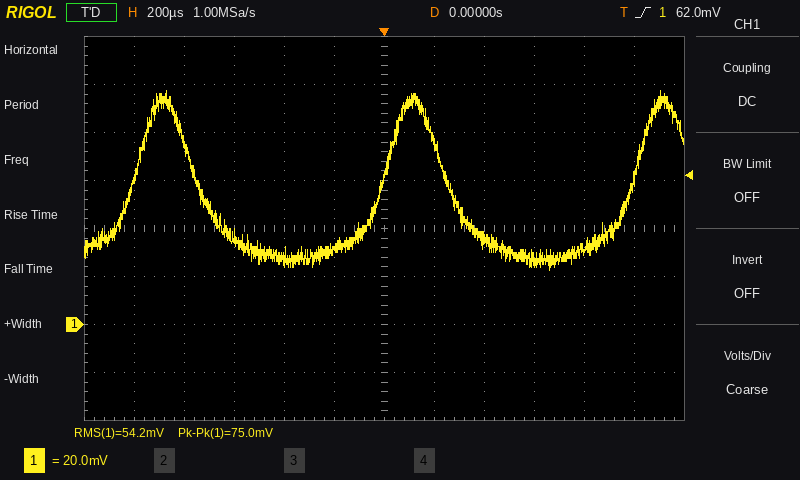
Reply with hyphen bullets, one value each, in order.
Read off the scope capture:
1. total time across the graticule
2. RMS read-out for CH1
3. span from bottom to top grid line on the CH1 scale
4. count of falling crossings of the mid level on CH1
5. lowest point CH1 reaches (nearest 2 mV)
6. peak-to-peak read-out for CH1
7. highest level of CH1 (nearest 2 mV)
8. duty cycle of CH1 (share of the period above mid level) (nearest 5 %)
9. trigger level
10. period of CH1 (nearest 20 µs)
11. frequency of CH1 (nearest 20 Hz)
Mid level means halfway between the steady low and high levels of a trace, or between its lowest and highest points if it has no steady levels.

- 2.4 ms
- 54.2 mV
- 160 mV
- 2
- 22 mV
- 75.0 mV
- 98 mV
- 25 %
- 62.0 mV
- 1.00 ms
- 1.00 kHz
